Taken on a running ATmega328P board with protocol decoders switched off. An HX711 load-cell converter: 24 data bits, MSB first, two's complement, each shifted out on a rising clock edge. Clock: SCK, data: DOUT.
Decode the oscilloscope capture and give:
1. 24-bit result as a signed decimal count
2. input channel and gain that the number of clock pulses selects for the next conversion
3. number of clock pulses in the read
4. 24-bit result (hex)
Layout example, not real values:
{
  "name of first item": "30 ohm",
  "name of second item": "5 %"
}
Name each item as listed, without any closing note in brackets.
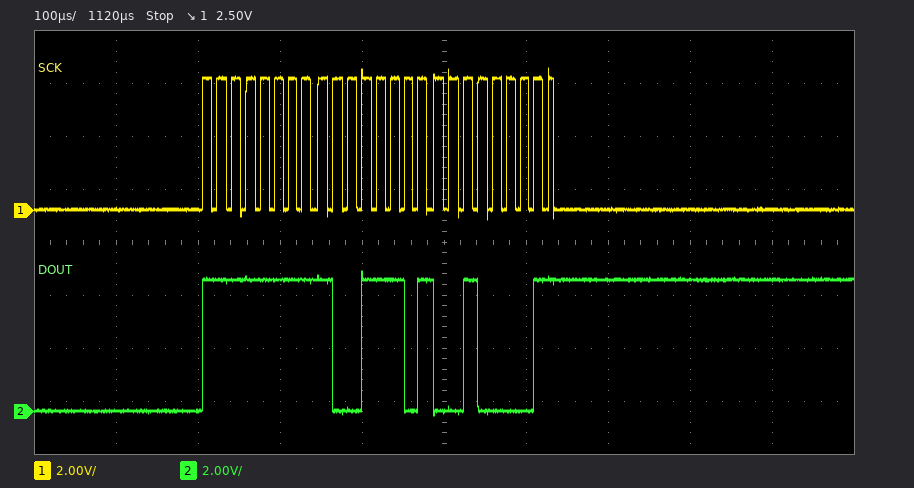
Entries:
{
  "24-bit result as a signed decimal count": "-25311",
  "input channel and gain that the number of clock pulses selects for the next conversion": "channel A, gain 128",
  "number of clock pulses in the read": "25",
  "24-bit result": "0xFF9D21"
}
